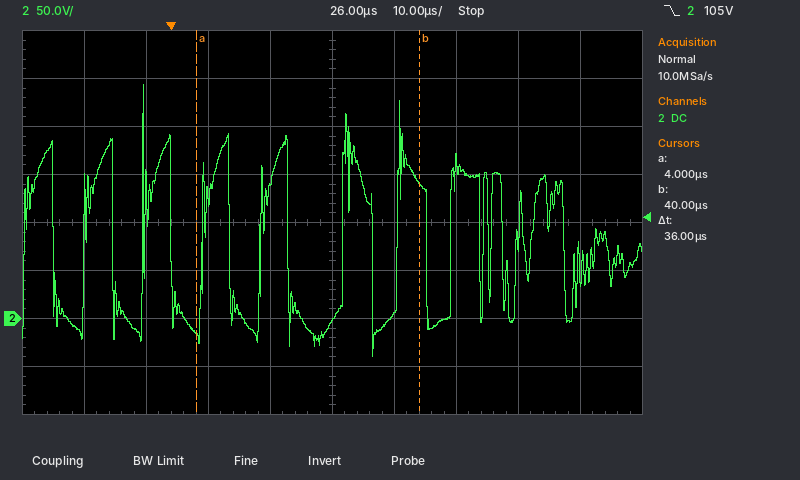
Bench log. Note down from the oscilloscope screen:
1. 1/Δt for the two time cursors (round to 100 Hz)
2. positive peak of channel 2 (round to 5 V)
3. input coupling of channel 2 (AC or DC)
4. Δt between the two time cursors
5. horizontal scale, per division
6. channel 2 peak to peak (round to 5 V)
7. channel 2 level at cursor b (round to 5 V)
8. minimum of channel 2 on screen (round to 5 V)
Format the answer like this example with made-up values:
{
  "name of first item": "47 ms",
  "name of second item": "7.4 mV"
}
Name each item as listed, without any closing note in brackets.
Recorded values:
{
  "1/Δt for the two time cursors": "27.8 kHz",
  "positive peak of channel 2": "245 V",
  "input coupling of channel 2": "DC",
  "Δt between the two time cursors": "36 µs",
  "horizontal scale, per division": "10 µs",
  "channel 2 peak to peak": "285 V",
  "channel 2 level at cursor b": "140 V",
  "minimum of channel 2 on screen": "-40 V"
}
